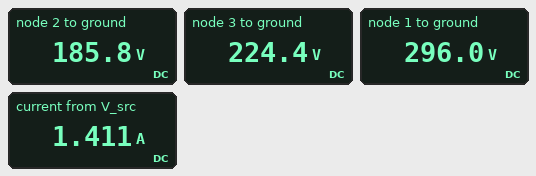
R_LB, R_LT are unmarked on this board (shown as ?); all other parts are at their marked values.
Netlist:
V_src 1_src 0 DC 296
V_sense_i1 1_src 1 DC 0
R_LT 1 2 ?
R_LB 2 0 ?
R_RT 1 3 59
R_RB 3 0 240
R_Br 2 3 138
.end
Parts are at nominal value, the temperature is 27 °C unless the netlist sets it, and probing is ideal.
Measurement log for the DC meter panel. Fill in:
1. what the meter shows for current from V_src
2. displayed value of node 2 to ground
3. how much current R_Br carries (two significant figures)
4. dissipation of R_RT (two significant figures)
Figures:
1.411 A
185.8 V
280 mA
87 W
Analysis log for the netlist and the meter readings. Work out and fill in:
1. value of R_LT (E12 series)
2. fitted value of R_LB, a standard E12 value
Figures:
560 Ω
390 Ω
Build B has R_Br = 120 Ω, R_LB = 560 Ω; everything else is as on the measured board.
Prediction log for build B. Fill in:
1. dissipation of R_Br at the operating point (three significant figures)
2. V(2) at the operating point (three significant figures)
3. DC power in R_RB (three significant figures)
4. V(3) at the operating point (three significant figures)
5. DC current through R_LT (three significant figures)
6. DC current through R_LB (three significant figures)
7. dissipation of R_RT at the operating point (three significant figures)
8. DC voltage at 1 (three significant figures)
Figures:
4.81 W
204 V
217 W
228 V
164 mA
364 mA
78.1 W
296 V
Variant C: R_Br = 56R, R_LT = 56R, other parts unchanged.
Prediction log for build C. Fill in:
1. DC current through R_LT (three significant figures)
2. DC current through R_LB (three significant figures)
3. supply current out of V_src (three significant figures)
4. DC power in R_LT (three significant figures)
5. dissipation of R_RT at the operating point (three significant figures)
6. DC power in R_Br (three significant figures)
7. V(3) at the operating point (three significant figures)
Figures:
786 mA
646 mA
1.66 A
34.6 W
45.5 W
1.09 W
244 V
